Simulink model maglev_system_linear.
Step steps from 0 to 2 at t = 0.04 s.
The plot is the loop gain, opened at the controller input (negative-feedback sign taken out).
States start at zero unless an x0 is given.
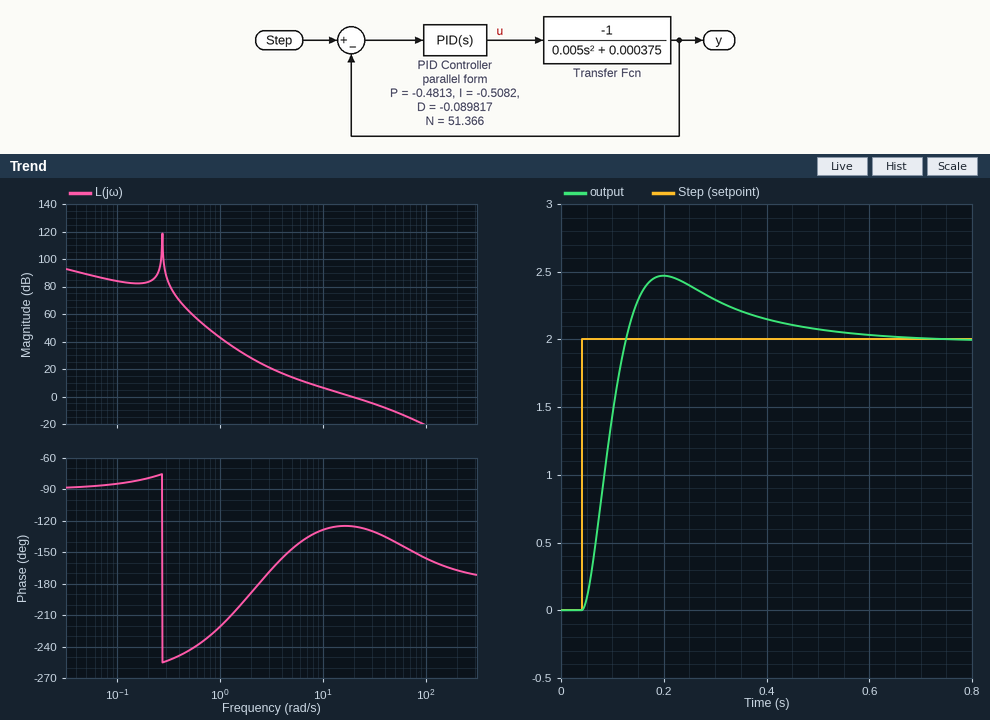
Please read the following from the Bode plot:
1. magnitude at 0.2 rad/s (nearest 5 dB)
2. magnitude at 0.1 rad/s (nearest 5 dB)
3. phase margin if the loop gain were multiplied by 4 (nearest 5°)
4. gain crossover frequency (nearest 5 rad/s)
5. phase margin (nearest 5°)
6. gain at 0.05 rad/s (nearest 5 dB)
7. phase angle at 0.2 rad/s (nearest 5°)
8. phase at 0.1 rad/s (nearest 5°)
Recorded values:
85 dB
85 dB
40°
20 rad/s
55°
90 dB
-80°
-85°
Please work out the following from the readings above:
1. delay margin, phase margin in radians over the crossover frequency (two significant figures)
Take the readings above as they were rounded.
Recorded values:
0.048 s
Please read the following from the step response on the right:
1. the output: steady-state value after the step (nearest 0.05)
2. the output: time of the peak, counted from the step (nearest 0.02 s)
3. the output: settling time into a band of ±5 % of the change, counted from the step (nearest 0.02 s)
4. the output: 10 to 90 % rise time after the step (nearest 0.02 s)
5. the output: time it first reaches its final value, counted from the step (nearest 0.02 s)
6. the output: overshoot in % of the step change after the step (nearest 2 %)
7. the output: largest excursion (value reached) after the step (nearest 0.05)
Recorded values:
2.00
0.16 s
0.42 s
0.06 s
0.08 s
24 %
2.45
